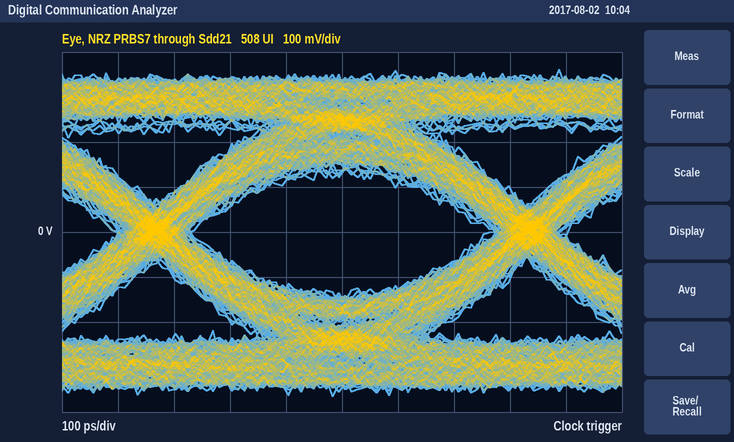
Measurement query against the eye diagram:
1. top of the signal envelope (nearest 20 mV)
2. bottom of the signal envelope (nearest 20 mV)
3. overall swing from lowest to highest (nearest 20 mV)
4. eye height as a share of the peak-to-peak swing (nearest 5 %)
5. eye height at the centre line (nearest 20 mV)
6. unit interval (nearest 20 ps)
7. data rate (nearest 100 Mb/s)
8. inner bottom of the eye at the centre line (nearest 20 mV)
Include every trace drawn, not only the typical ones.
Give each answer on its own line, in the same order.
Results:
360 mV
-360 mV
720 mV
40 %
280 mV
660 ps
1.5 Gb/s
-140 mV
